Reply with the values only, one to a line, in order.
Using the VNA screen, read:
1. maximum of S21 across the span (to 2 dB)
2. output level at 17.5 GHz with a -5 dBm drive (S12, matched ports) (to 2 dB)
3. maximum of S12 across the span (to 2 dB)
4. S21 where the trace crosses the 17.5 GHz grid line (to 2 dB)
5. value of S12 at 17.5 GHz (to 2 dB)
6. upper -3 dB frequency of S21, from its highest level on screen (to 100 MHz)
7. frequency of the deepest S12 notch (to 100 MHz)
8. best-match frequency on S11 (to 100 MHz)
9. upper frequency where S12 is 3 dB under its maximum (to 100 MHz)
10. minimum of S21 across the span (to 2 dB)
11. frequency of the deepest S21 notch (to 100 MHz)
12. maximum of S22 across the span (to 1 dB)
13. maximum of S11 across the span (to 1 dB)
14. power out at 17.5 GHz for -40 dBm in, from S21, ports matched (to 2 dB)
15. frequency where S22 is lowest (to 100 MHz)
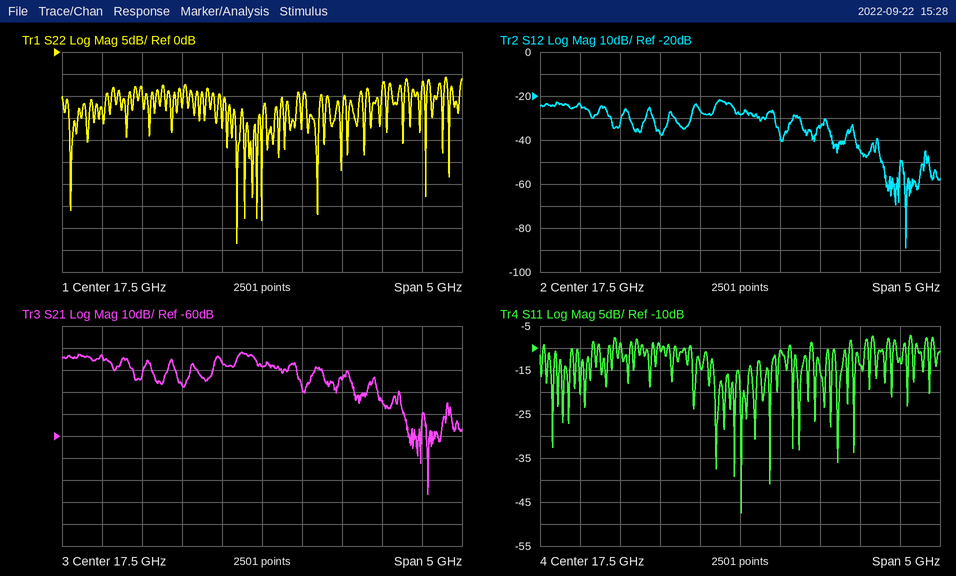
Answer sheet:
-22 dB
-34 dBm
-22 dB
-28 dB
-28 dB
17.4 GHz
19.6 GHz
17.5 GHz
17.4 GHz
-86 dB
19.6 GHz
-6 dB
-7 dB
-68 dBm
17.2 GHz
